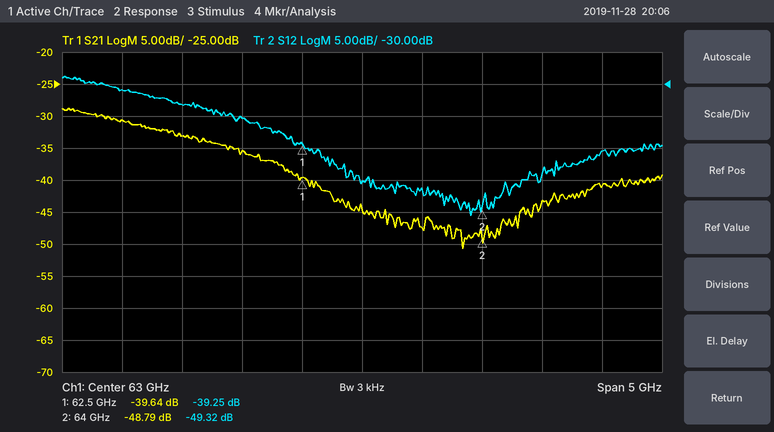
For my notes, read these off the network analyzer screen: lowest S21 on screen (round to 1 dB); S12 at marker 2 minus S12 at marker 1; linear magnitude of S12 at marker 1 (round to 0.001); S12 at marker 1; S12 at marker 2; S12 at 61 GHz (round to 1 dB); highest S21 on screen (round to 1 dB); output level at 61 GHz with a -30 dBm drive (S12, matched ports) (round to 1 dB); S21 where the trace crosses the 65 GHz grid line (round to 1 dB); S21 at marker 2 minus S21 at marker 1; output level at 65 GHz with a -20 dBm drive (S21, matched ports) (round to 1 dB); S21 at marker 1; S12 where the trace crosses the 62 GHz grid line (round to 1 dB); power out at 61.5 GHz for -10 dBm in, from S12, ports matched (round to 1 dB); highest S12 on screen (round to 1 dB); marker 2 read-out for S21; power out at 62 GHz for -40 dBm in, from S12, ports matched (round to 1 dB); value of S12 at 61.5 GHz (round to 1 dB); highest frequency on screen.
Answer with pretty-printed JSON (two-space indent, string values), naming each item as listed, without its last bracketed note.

{
  "lowest S21 on screen": "-51 dB",
  "S12 at marker 2 minus S12 at marker 1": "-10.07 dB",
  "linear magnitude of S12 at marker 1": "0.011",
  "S12 at marker 1": "-39.25 dB",
  "S12 at marker 2": "-49.32 dB",
  "S12 at 61 GHz": "-31 dB",
  "highest S21 on screen": "-29 dB",
  "output level at 61 GHz with a -30 dBm drive (S12, matched ports)": "-61 dBm",
  "S21 where the trace crosses the 65 GHz grid line": "-41 dB",
  "S21 at marker 2 minus S21 at marker 1": "-9.15 dB",
  "output level at 65 GHz with a -20 dBm drive (S21, matched ports)": "-61 dBm",
  "S21 at marker 1": "-39.64 dB",
  "S12 where the trace crosses the 62 GHz grid line": "-35 dB",
  "power out at 61.5 GHz for -10 dBm in, from S12, ports matched": "-43 dBm",
  "highest S12 on screen": "-29 dB",
  "marker 2 read-out for S21": "-48.79 dB",
  "power out at 62 GHz for -40 dBm in, from S12, ports matched": "-75 dBm",
  "value of S12 at 61.5 GHz": "-33 dB",
  "highest frequency on screen": "65.5 GHz"
}
